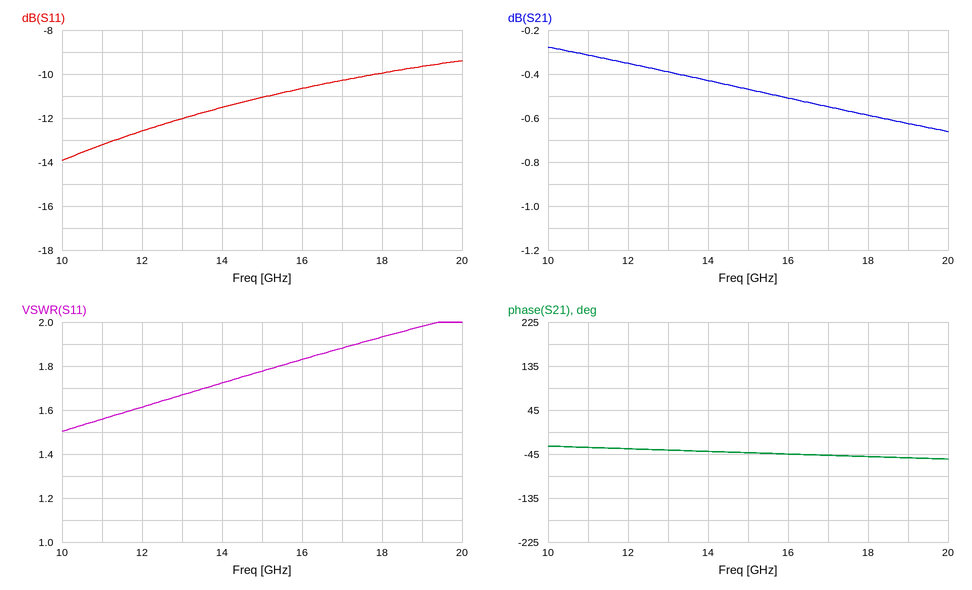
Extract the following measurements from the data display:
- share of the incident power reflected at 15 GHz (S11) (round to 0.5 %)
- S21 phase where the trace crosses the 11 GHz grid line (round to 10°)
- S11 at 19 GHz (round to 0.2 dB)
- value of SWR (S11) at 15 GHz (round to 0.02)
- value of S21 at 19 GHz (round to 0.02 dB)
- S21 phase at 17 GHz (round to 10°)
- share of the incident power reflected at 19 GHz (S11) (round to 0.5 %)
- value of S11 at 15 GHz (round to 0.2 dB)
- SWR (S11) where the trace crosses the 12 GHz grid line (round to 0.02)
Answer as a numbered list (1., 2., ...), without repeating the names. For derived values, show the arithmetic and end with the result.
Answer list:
1. 10^(-11/10) ≈ 7.94 %, so 8.0 % to the nearest 0.5 %
2. -30°
3. -9.6 dB
4. 1.78
5. -0.62 dB
6. -50°
7. 10^(-9.6/10) ≈ 11.0 %
8. -11.0 dB
9. 1.62
